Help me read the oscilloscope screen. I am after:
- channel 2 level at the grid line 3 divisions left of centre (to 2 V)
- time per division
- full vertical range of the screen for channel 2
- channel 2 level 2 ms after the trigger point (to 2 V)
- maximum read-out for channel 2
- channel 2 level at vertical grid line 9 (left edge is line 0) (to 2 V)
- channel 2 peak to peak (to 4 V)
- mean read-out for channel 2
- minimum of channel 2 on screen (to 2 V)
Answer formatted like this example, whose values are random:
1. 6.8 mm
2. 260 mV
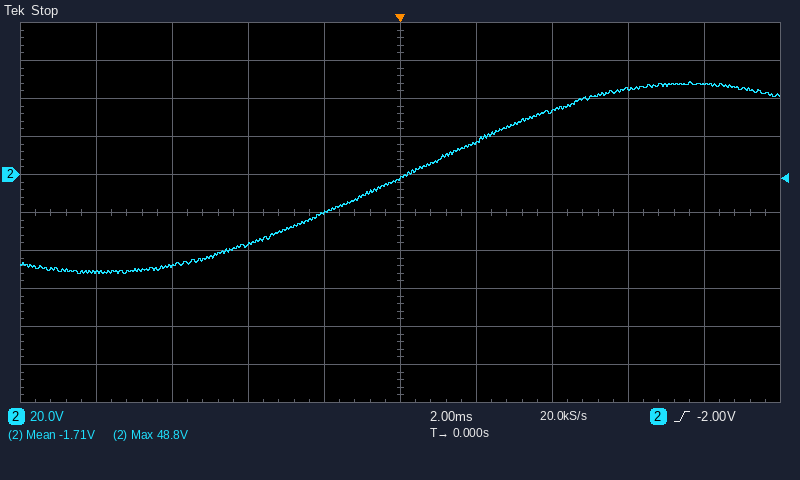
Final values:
1. -48 V
2. 2 ms
3. 200 V
4. 18 V
5. 48.8 V
6. 48 V
7. 100 V
8. -1.71 V
9. -52 V
